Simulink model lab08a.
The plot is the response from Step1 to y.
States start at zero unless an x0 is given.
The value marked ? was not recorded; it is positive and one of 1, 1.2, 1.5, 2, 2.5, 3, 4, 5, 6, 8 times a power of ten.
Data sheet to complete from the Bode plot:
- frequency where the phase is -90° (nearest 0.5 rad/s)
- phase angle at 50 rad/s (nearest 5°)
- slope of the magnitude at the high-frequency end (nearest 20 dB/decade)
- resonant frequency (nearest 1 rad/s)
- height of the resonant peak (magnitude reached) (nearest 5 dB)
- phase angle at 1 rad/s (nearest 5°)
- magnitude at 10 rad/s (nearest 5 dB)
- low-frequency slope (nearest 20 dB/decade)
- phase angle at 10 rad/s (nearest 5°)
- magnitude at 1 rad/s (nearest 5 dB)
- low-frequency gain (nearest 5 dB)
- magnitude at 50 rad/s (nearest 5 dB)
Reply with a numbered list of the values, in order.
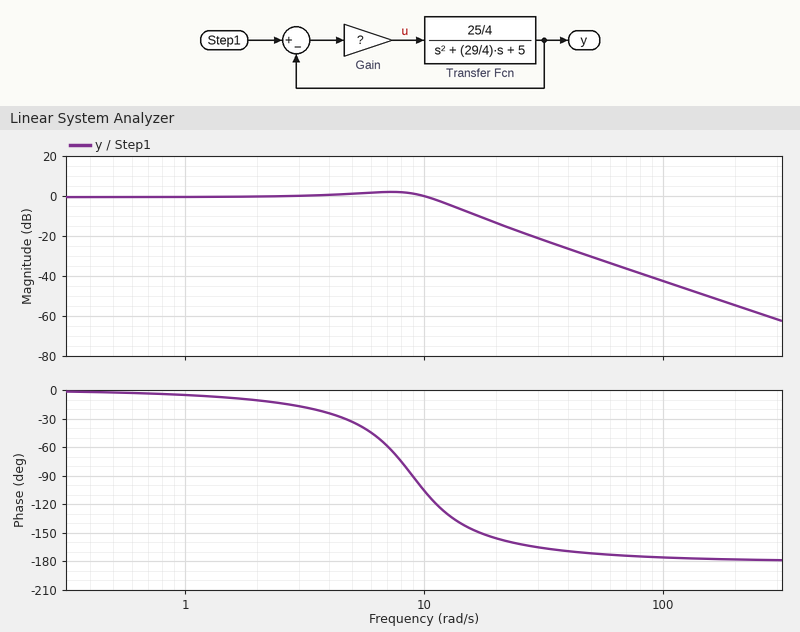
1. 9.0 rad/s
2. -170°
3. -40 dB/decade
4. 7 rad/s
5. 0 dB
6. -5°
7. 0 dB
8. 0 dB/decade
9. -105°
10. 0 dB
11. 0 dB
12. -30 dB
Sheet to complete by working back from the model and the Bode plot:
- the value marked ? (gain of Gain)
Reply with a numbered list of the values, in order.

1. 12
